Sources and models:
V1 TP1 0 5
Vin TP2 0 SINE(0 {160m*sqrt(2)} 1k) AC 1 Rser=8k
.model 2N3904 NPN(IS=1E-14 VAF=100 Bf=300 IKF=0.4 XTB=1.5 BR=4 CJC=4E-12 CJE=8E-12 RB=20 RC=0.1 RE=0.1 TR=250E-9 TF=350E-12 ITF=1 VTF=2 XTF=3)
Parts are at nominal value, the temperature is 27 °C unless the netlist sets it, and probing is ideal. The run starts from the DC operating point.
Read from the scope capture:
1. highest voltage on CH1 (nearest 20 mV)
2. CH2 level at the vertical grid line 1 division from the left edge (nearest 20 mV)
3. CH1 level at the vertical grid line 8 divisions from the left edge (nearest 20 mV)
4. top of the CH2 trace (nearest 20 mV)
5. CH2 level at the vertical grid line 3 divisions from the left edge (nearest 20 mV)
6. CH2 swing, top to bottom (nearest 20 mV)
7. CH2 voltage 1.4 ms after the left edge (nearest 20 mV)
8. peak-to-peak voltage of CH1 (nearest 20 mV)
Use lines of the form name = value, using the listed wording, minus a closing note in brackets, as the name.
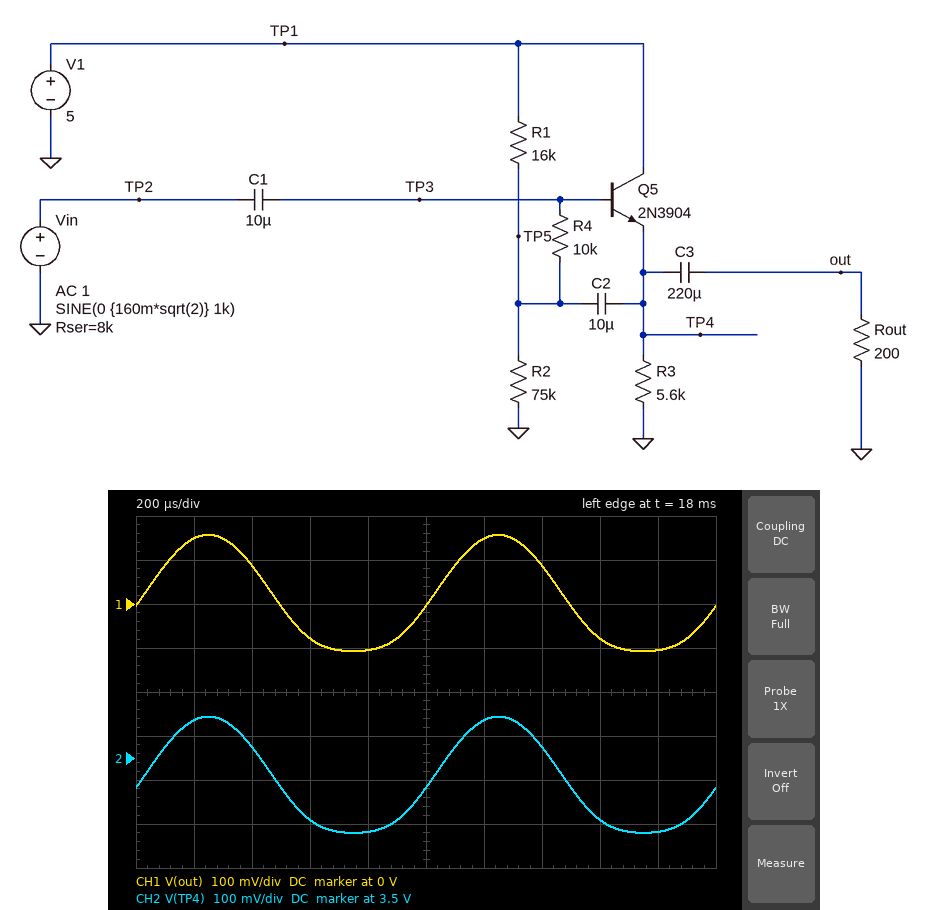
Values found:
highest voltage on CH1 = 160 mV
CH2 level at the vertical grid line 1 division from the left edge = 3.58 V
CH1 level at the vertical grid line 8 divisions from the left edge = -80 mV
top of the CH2 trace = 3.60 V
CH2 level at the vertical grid line 3 divisions from the left edge = 3.36 V
CH2 swing, top to bottom = 260 mV
CH2 voltage 1.4 ms after the left edge = 3.52 V
peak-to-peak voltage of CH1 = 260 mV
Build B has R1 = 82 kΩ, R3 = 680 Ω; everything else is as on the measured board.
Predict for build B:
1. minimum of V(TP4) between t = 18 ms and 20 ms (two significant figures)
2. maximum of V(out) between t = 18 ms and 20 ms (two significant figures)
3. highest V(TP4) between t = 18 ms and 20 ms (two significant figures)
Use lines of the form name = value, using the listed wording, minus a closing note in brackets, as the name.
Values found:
minimum of V(TP4) between t = 18 ms and 20 ms = 1.2 V
maximum of V(out) between t = 18 ms and 20 ms = 170 mV
highest V(TP4) between t = 18 ms and 20 ms = 1.6 V
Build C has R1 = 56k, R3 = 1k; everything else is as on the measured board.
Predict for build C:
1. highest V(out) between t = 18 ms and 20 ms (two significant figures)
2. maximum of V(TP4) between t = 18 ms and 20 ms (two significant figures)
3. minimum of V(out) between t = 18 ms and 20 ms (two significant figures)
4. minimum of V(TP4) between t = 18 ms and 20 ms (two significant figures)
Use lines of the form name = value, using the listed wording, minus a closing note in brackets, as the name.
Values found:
highest V(out) between t = 18 ms and 20 ms = 180 mV
maximum of V(TP4) between t = 18 ms and 20 ms = 2.1 V
minimum of V(out) between t = 18 ms and 20 ms = -170 mV
minimum of V(TP4) between t = 18 ms and 20 ms = 1.8 V
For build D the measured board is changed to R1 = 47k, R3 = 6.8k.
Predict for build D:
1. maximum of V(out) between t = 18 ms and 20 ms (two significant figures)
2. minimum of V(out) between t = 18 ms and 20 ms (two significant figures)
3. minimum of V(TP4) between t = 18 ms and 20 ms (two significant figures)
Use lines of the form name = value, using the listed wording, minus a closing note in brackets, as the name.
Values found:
maximum of V(out) between t = 18 ms and 20 ms = 140 mV
minimum of V(out) between t = 18 ms and 20 ms = -68 mV
minimum of V(TP4) between t = 18 ms and 20 ms = 2.3 V
